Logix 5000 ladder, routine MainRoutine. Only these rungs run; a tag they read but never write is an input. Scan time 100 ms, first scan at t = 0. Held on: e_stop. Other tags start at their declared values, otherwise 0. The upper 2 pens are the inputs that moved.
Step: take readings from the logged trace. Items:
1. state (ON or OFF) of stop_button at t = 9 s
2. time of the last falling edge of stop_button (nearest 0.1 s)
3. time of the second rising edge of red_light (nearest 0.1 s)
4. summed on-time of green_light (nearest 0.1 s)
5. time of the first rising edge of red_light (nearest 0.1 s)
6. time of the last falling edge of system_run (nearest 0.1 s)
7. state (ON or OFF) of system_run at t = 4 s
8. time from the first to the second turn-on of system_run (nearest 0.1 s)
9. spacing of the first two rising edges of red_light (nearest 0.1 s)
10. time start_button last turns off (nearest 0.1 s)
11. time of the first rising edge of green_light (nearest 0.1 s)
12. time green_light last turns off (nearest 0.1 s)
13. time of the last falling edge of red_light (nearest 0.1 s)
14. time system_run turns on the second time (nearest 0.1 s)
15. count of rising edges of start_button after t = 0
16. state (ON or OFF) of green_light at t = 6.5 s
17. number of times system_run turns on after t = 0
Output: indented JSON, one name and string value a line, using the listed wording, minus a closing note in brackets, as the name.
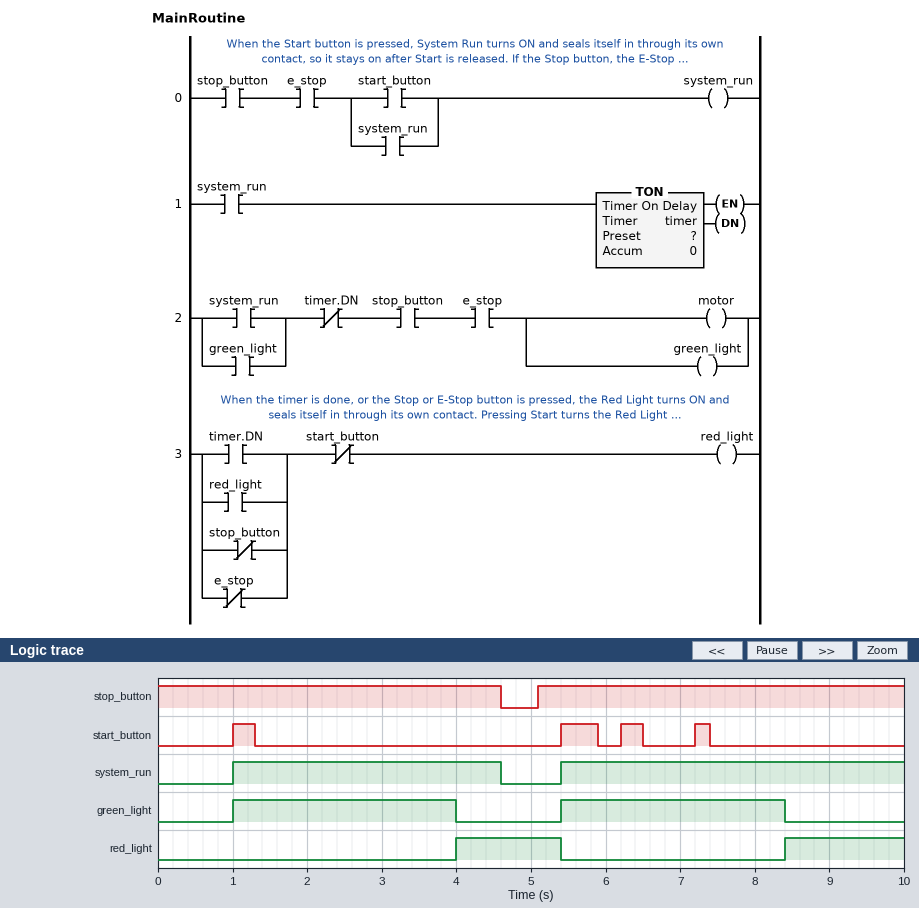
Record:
{
  "state (ON or OFF) of stop_button at t = 9 s": "ON",
  "time of the last falling edge of stop_button": "4.6 s",
  "time of the second rising edge of red_light": "8.4 s",
  "summed on-time of green_light": "6.0 s",
  "time of the first rising edge of red_light": "4.0 s",
  "time of the last falling edge of system_run": "4.6 s",
  "state (ON or OFF) of system_run at t = 4 s": "ON",
  "time from the first to the second turn-on of system_run": "4.4 s",
  "spacing of the first two rising edges of red_light": "4.4 s",
  "time start_button last turns off": "7.4 s",
  "time of the first rising edge of green_light": "1.0 s",
  "time green_light last turns off": "8.4 s",
  "time of the last falling edge of red_light": "5.4 s",
  "time system_run turns on the second time": "5.4 s",
  "count of rising edges of start_button after t = 0": "4",
  "state (ON or OFF) of green_light at t = 6.5 s": "ON",
  "number of times system_run turns on after t = 0": "2"
}
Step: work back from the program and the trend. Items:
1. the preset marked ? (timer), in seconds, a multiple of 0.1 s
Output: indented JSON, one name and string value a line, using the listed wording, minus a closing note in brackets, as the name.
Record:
{
  "the preset marked ? (timer), in seconds, a multiple of 0.1 s": "3.0 s"
}
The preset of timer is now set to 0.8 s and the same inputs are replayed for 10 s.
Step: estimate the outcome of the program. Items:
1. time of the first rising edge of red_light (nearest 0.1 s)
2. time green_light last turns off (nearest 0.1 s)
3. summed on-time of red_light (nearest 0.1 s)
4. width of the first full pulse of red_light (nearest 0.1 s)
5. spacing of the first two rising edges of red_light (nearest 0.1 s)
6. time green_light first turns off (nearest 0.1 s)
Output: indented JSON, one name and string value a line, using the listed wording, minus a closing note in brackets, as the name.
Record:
{
  "time of the first rising edge of red_light": "1.8 s",
  "time green_light last turns off": "6.2 s",
  "summed on-time of red_light": "6.9 s",
  "width of the first full pulse of red_light": "3.6 s",
  "spacing of the first two rising edges of red_light": "4.7 s",
  "time green_light first turns off": "1.8 s"
}
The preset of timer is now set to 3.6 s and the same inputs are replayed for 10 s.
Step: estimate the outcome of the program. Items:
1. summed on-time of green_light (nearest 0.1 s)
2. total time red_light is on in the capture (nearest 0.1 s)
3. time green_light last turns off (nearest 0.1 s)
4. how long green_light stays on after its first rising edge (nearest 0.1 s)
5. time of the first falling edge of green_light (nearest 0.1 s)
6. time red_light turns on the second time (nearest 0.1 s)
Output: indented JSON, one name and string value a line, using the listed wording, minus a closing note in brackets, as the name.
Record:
{
  "summed on-time of green_light": "7.2 s",
  "total time red_light is on in the capture": "1.8 s",
  "time green_light last turns off": "9.0 s",
  "how long green_light stays on after its first rising edge": "3.6 s",
  "time of the first falling edge of green_light": "4.6 s",
  "time red_light turns on the second time": "9.0 s"
}
